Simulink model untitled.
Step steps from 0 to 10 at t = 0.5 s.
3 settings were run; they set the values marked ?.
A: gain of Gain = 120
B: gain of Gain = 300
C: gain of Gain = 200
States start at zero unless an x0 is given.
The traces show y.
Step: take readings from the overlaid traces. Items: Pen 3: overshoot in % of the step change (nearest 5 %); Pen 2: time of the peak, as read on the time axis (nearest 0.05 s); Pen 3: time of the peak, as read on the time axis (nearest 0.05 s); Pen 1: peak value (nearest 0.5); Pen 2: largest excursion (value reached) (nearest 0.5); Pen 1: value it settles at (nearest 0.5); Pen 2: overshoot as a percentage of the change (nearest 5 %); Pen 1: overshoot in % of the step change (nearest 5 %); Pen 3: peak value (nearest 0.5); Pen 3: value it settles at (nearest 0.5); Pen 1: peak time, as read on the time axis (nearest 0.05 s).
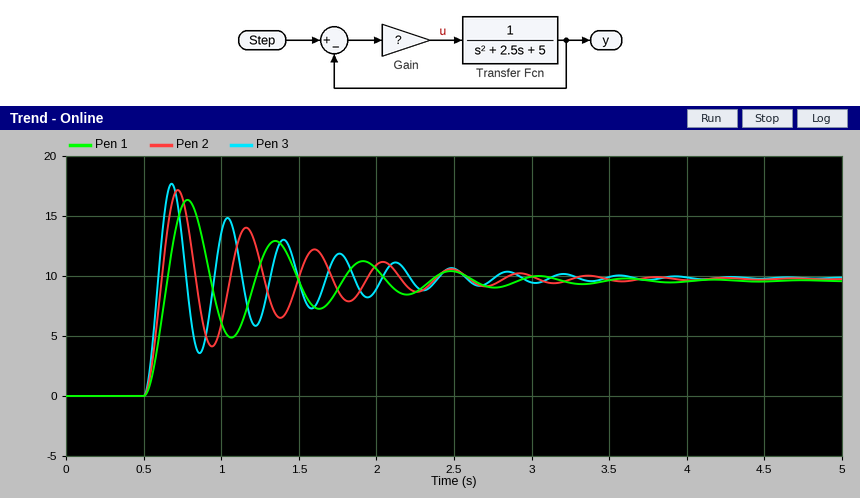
80 %
0.70 s
0.70 s
16.5
17.0
9.5
75 %
70 %
17.5
10.0
0.80 s
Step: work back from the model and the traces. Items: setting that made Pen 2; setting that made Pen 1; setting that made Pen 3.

C
A
B
